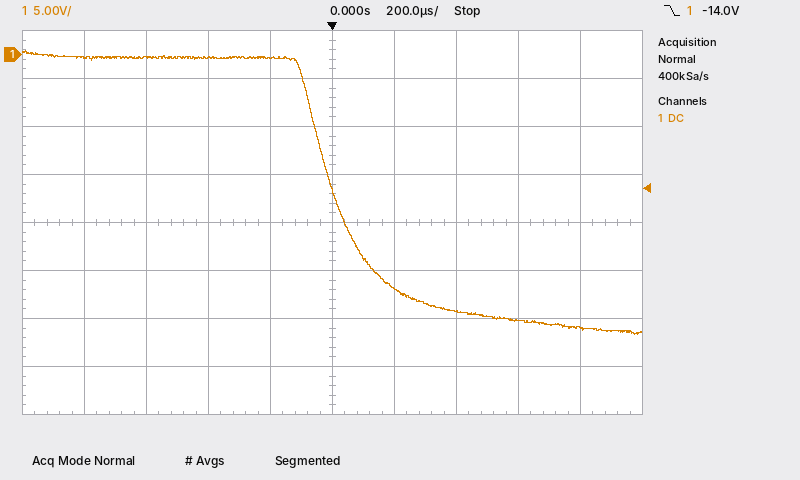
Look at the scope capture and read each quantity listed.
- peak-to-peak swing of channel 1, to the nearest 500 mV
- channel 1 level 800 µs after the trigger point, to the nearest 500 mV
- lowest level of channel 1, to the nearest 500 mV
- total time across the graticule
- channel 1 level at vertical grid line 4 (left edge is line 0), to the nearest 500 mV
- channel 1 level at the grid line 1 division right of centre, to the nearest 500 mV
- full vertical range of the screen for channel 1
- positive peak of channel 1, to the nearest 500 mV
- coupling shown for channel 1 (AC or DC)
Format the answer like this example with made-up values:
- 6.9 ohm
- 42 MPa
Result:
- 29.5 V
- -28.5 V
- -29.0 V
- 2 ms
- -500 mV
- -24.5 V
- 40 V
- 500 mV
- DC
